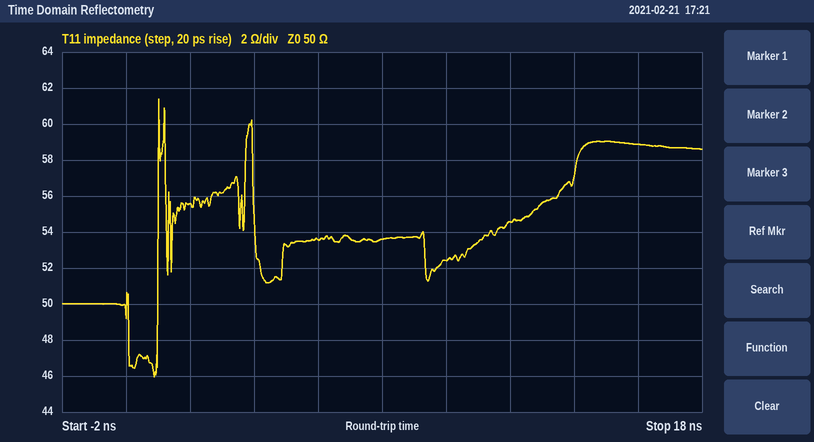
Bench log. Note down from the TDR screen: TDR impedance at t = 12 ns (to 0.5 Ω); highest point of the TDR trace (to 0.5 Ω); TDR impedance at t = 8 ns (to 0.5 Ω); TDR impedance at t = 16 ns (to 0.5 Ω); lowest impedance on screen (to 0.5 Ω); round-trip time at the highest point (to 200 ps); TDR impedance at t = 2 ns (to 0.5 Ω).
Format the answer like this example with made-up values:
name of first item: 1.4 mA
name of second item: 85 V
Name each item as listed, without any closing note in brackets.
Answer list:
TDR impedance at t = 12 ns: 54.5 Ω
highest point of the TDR trace: 61.5 Ω
TDR impedance at t = 8 ns: 53.5 Ω
TDR impedance at t = 16 ns: 59.0 Ω
lowest impedance on screen: 46.0 Ω
round-trip time at the highest point: 1.0 ns
TDR impedance at t = 2 ns: 55.5 Ω
